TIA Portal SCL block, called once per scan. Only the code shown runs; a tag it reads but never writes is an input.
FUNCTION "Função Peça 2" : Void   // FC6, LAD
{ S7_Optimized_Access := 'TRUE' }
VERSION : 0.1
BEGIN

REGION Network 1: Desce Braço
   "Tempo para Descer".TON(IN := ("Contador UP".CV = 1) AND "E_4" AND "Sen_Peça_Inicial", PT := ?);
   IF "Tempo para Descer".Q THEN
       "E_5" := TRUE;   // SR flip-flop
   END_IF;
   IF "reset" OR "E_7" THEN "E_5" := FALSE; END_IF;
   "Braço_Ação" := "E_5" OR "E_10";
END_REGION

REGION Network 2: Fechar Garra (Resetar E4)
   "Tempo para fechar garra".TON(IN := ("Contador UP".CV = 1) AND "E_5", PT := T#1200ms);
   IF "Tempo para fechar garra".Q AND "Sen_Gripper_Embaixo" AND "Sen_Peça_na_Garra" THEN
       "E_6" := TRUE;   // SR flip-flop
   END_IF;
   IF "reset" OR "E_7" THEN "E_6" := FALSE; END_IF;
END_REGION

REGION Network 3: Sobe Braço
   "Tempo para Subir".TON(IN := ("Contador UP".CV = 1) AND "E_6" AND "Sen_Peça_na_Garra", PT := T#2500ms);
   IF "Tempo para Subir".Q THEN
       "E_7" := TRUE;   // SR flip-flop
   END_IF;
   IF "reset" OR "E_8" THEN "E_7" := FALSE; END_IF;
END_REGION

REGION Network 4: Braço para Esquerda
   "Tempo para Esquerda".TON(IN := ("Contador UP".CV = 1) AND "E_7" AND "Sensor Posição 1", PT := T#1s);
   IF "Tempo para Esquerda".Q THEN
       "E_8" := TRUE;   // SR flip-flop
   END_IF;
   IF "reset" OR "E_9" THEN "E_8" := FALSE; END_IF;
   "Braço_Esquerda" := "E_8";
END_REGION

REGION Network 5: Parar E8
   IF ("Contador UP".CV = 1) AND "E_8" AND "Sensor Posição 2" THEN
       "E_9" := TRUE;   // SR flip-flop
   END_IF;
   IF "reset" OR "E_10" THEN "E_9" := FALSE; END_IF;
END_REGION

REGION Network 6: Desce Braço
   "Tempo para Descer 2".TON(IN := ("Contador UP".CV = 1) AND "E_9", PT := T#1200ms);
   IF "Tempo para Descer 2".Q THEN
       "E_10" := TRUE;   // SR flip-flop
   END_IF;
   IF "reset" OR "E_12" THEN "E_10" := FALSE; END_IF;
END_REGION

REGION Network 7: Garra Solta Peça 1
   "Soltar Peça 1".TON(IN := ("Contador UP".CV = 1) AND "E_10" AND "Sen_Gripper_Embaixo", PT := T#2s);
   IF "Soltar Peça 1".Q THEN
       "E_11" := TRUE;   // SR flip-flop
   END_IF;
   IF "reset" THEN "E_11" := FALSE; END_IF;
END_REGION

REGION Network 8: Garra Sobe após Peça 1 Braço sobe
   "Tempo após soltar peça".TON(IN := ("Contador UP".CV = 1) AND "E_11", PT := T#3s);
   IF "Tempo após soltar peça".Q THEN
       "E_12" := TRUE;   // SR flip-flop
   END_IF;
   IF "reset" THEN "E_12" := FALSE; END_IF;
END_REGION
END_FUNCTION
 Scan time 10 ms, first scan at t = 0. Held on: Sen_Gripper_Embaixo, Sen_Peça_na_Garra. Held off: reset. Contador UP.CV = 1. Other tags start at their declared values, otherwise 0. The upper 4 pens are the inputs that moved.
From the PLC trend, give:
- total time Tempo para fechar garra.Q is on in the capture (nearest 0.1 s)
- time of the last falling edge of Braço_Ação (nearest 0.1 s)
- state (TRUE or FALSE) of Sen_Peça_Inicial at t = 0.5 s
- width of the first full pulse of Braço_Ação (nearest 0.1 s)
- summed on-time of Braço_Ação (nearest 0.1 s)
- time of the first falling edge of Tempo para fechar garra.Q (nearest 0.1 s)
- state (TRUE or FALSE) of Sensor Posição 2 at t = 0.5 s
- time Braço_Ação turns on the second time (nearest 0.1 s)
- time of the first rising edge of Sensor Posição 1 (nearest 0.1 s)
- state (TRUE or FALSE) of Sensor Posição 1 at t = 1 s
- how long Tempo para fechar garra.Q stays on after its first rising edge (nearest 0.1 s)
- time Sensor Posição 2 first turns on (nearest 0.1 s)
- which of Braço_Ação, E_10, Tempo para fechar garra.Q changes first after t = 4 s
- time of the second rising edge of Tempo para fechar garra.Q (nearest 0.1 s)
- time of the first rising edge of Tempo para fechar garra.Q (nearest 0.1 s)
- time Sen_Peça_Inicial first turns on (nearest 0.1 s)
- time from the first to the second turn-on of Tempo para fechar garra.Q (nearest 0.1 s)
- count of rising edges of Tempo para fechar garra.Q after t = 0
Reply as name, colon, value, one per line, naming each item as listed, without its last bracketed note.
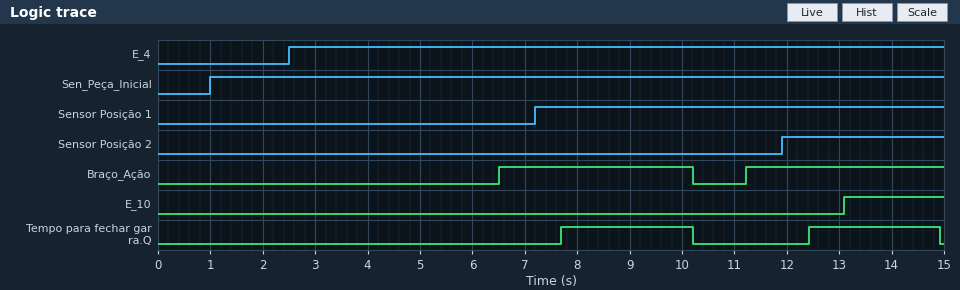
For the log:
total time Tempo para fechar garra.Q is on in the capture: 5.0 s
time of the last falling edge of Braço_Ação: 10.2 s
state (TRUE or FALSE) of Sen_Peça_Inicial at t = 0.5 s: FALSE
width of the first full pulse of Braço_Ação: 3.7 s
summed on-time of Braço_Ação: 7.5 s
time of the first falling edge of Tempo para fechar garra.Q: 10.2 s
state (TRUE or FALSE) of Sensor Posição 2 at t = 0.5 s: FALSE
time Braço_Ação turns on the second time: 11.2 s
time of the first rising edge of Sensor Posição 1: 7.2 s
state (TRUE or FALSE) of Sensor Posição 1 at t = 1 s: FALSE
how long Tempo para fechar garra.Q stays on after its first rising edge: 2.5 s
time Sensor Posição 2 first turns on: 11.9 s
which of Braço_Ação, E_10, Tempo para fechar garra.Q changes first after t = 4 s: Braço_Ação
time of the second rising edge of Tempo para fechar garra.Q: 12.4 s
time of the first rising edge of Tempo para fechar garra.Q: 7.7 s
time Sen_Peça_Inicial first turns on: 1.0 s
time from the first to the second turn-on of Tempo para fechar garra.Q: 4.7 s
count of rising edges of Tempo para fechar garra.Q after t = 0: 2
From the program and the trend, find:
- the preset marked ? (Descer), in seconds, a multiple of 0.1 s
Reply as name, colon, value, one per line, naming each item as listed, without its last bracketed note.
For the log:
the preset marked ? (Descer), in seconds, a multiple of 0.1 s: 4.0 s
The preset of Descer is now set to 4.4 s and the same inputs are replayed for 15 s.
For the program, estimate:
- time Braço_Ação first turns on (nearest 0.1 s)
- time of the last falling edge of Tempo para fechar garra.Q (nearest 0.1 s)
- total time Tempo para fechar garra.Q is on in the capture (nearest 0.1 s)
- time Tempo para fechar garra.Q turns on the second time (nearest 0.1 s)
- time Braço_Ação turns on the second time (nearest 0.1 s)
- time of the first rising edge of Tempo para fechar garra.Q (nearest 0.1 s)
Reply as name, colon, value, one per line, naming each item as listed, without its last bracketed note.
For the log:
time Braço_Ação first turns on: 6.9 s
time of the last falling edge of Tempo para fechar garra.Q: 10.6 s
total time Tempo para fechar garra.Q is on in the capture: 4.7 s
time Tempo para fechar garra.Q turns on the second time: 12.8 s
time Braço_Ação turns on the second time: 11.6 s
time of the first rising edge of Tempo para fechar garra.Q: 8.1 s
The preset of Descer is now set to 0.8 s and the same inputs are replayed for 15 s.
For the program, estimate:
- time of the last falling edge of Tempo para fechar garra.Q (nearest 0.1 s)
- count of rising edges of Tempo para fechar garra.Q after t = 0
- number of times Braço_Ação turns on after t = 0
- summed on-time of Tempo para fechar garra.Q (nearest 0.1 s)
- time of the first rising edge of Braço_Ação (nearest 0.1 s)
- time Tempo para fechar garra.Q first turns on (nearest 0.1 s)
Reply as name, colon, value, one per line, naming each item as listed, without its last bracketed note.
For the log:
time of the last falling edge of Tempo para fechar garra.Q: 11.9 s
count of rising edges of Tempo para fechar garra.Q after t = 0: 3
number of times Braço_Ação turns on after t = 0: 3
summed on-time of Tempo para fechar garra.Q: 5.7 s
time of the first rising edge of Braço_Ação: 3.3 s
time Tempo para fechar garra.Q first turns on: 4.5 s
